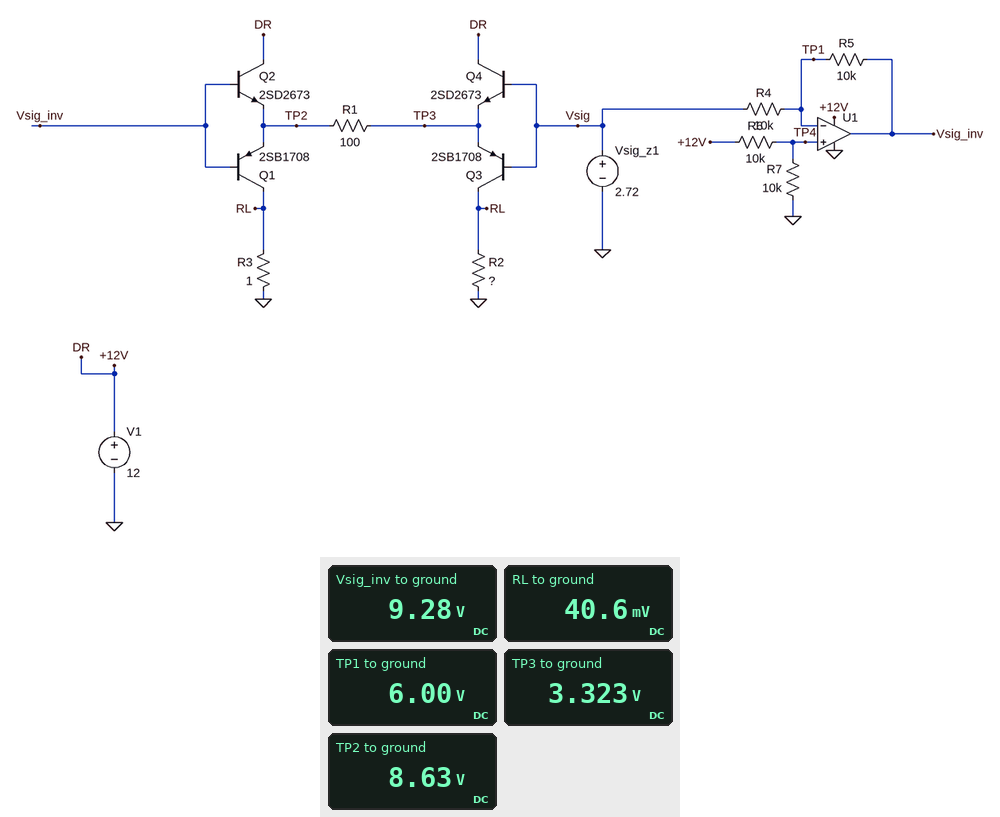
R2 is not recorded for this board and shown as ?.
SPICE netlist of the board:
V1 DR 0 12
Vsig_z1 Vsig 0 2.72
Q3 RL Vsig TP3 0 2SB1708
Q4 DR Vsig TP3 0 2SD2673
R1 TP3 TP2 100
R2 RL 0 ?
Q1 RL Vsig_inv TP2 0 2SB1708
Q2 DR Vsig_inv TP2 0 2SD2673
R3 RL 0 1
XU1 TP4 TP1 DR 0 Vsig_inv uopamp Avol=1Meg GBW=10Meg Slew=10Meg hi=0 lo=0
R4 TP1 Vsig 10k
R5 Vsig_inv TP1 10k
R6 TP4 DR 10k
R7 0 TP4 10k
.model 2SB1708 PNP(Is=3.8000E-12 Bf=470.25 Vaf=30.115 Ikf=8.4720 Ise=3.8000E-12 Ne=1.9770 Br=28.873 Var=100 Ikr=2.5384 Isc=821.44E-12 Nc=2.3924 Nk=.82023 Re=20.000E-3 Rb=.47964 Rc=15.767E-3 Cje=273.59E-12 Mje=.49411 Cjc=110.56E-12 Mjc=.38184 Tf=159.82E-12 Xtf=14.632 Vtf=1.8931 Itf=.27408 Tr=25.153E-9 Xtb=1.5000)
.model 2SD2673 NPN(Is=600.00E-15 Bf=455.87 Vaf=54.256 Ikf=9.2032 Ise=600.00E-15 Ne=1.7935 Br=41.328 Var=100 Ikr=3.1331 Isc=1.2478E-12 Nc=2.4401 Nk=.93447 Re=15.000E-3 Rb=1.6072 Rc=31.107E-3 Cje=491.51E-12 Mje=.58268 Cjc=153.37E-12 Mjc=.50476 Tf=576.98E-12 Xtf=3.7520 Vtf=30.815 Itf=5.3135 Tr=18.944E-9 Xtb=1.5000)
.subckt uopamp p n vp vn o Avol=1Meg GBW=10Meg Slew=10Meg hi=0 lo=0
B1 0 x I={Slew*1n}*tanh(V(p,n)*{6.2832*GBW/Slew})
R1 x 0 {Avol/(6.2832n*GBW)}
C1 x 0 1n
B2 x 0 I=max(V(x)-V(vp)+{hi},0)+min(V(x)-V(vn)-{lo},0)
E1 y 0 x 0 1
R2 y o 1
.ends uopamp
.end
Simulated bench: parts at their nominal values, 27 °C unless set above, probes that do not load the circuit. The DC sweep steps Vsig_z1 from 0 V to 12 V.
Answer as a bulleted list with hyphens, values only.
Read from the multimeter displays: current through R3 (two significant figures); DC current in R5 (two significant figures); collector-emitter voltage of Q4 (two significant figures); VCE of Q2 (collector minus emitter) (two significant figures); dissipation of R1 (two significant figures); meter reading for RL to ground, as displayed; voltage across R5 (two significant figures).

- 41 mA
- 330 µA
- 8.7 V
- 3.4 V
- 280 mW
- 40.6 mV
- 3.3 V
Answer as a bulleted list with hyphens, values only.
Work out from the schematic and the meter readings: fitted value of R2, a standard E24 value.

- 3.3 Ω
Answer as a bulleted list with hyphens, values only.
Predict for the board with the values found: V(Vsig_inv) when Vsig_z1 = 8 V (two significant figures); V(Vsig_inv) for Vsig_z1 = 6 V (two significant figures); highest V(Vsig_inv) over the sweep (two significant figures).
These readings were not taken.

- 4.0 V
- 6.0 V
- 12 V
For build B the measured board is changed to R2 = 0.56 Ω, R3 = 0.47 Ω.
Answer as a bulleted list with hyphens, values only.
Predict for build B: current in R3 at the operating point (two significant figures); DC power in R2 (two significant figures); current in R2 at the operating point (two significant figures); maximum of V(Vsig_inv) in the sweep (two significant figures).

- 29 mA
- 330 µW
- 24 mA
- 12 V
